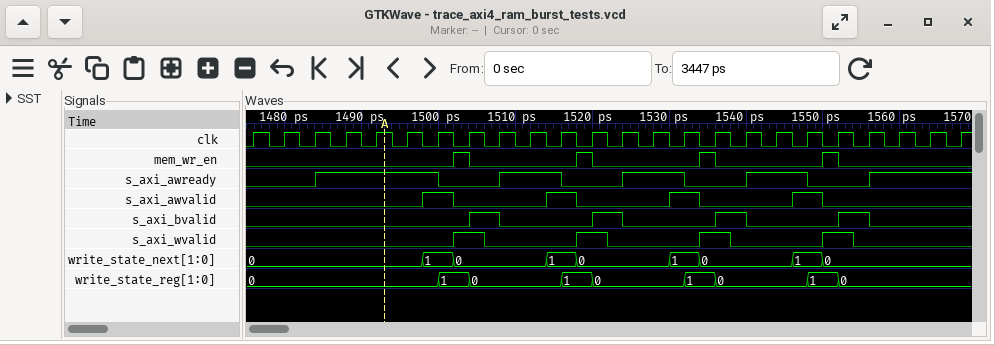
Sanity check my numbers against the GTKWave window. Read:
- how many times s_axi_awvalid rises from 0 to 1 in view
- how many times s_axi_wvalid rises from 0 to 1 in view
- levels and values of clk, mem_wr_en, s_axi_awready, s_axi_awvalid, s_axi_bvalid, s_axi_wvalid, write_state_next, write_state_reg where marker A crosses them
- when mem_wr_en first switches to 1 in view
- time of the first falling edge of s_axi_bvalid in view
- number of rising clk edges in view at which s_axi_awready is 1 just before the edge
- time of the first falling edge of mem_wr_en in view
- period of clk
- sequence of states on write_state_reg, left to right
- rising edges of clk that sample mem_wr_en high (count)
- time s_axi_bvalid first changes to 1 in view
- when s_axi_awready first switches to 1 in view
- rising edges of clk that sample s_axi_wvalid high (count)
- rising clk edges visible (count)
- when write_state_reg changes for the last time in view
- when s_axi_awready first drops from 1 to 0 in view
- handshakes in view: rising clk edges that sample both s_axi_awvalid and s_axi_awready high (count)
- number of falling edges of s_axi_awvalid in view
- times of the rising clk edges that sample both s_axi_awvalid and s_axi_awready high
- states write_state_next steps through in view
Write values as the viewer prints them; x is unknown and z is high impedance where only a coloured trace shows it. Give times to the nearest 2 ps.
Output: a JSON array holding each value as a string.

["4", "4", "clk=1, mem_wr_en=0, s_axi_awready=1, s_axi_awvalid=0, s_axi_bvalid=0, s_axi_wvalid=0, write_state_next=0, write_state_reg=0", "1502 ps", "1508 ps", "13", "1504 ps", "4 ps", "0, 1, 0, 1, 0, 1, 0, 1, 0", "4", "1504 ps", "1484 ps", "4", "24", "1552 ps", "1500 ps", "4", "4", "1500 ps, 1516 ps, 1532 ps, 1548 ps", "0, 1, 0, 1, 0, 1, 0, 1, 0"]
